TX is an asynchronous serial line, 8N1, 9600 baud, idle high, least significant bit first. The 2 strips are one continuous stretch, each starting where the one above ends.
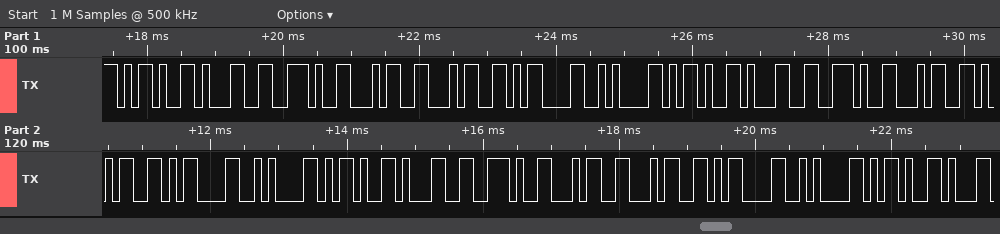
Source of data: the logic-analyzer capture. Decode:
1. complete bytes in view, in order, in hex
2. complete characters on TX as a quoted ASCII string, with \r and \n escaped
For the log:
0x2D 0x31 0x2E 0x34 0x34 0x0D 0x0A 0x2D 0x31 0x2E 0x34 0x35 0x0D 0x0A 0x2D 0x31 0x2E 0x34 0x34 0x0D 0x0A 0x2D
"-1.44\r\n-1.45\r\n-1.44\r\n-"
